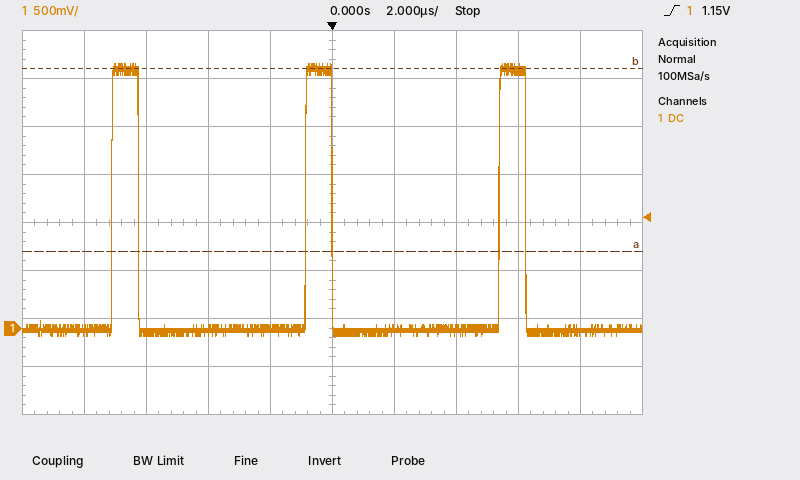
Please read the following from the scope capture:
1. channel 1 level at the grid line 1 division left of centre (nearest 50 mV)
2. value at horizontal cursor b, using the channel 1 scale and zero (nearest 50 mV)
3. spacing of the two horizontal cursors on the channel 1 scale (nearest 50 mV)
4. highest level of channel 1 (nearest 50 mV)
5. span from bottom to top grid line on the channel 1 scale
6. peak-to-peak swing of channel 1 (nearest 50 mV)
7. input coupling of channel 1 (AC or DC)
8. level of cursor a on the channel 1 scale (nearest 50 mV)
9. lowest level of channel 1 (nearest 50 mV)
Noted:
0 mV
2.70 V
1.90 V
2.75 V
4 V
2.85 V
DC
800 mV
-100 mV
